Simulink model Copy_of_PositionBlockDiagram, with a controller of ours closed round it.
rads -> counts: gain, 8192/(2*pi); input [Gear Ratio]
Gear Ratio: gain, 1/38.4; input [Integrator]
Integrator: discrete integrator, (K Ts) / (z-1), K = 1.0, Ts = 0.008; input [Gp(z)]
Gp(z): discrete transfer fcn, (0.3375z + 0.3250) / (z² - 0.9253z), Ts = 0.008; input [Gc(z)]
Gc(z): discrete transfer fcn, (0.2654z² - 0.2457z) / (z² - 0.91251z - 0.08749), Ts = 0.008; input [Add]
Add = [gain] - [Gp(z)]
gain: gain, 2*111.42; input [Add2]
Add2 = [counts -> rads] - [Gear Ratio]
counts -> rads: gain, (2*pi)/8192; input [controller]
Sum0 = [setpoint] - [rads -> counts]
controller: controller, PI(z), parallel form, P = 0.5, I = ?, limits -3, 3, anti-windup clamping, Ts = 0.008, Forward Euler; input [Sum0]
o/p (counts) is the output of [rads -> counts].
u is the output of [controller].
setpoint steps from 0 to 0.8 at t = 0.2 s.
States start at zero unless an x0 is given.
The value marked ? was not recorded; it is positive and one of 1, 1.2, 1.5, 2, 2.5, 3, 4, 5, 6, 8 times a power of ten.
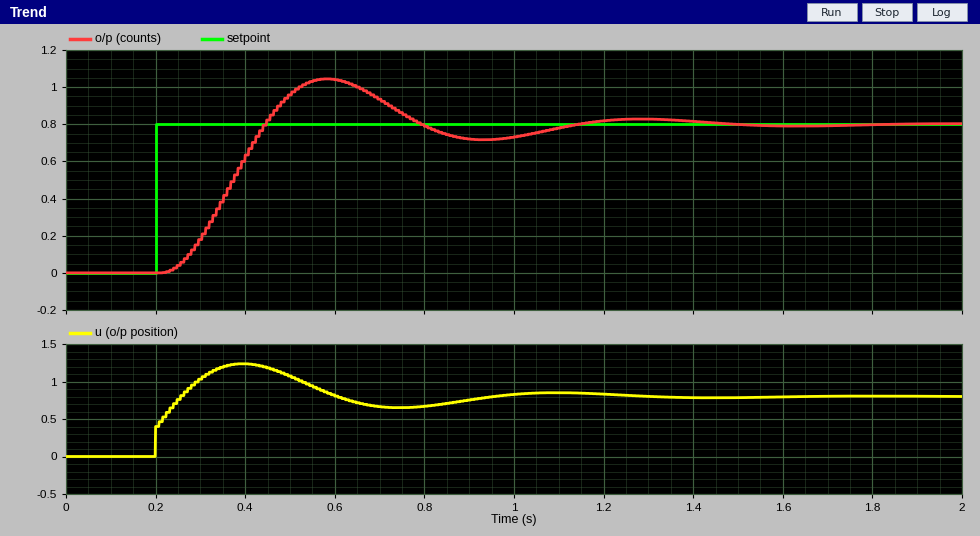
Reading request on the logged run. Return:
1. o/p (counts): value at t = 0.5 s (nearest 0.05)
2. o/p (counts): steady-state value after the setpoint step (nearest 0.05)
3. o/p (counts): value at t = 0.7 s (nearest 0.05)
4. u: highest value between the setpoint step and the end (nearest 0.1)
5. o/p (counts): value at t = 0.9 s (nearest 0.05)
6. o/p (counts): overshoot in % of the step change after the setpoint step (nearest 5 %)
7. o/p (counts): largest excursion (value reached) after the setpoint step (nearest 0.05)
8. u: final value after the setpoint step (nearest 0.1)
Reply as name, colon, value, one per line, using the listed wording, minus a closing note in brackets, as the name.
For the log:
o/p (counts): value at t = 0.5 s: 0.95
o/p (counts): steady-state value after the setpoint step: 0.80
o/p (counts): value at t = 0.7 s: 0.95
u: highest value between the setpoint step and the end: 1.2
o/p (counts): value at t = 0.9 s: 0.70
o/p (counts): overshoot in % of the step change after the setpoint step: 30 %
o/p (counts): largest excursion (value reached) after the setpoint step: 1.05
u: final value after the setpoint step: 0.8
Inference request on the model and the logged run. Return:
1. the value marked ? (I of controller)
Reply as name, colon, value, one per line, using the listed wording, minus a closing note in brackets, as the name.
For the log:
the value marked ?: 10
